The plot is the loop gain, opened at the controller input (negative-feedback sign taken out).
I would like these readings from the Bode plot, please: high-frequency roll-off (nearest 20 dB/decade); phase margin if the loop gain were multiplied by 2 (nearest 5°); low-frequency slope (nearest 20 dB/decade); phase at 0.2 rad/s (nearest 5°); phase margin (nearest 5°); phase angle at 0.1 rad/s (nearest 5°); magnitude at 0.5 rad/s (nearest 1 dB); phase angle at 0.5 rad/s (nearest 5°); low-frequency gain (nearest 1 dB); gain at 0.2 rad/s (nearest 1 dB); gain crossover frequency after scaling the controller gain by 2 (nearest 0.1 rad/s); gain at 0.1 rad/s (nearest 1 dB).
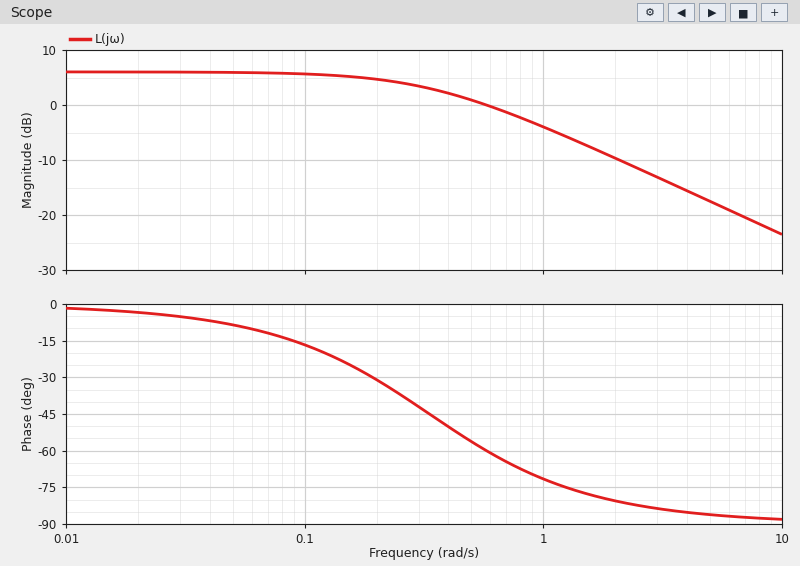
-20 dB/decade
105°
0 dB/decade
-30°
120°
-15°
1 dB
-55°
6 dB
5 dB
1.3 rad/s
6 dB
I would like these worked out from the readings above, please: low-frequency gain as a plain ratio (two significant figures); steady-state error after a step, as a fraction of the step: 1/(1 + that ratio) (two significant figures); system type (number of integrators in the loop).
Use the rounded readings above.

2.0
0.33
0
